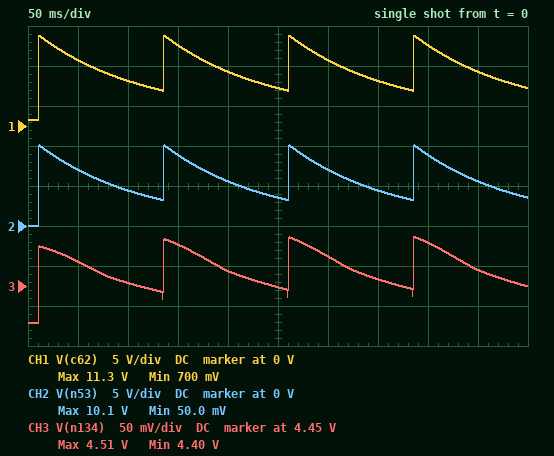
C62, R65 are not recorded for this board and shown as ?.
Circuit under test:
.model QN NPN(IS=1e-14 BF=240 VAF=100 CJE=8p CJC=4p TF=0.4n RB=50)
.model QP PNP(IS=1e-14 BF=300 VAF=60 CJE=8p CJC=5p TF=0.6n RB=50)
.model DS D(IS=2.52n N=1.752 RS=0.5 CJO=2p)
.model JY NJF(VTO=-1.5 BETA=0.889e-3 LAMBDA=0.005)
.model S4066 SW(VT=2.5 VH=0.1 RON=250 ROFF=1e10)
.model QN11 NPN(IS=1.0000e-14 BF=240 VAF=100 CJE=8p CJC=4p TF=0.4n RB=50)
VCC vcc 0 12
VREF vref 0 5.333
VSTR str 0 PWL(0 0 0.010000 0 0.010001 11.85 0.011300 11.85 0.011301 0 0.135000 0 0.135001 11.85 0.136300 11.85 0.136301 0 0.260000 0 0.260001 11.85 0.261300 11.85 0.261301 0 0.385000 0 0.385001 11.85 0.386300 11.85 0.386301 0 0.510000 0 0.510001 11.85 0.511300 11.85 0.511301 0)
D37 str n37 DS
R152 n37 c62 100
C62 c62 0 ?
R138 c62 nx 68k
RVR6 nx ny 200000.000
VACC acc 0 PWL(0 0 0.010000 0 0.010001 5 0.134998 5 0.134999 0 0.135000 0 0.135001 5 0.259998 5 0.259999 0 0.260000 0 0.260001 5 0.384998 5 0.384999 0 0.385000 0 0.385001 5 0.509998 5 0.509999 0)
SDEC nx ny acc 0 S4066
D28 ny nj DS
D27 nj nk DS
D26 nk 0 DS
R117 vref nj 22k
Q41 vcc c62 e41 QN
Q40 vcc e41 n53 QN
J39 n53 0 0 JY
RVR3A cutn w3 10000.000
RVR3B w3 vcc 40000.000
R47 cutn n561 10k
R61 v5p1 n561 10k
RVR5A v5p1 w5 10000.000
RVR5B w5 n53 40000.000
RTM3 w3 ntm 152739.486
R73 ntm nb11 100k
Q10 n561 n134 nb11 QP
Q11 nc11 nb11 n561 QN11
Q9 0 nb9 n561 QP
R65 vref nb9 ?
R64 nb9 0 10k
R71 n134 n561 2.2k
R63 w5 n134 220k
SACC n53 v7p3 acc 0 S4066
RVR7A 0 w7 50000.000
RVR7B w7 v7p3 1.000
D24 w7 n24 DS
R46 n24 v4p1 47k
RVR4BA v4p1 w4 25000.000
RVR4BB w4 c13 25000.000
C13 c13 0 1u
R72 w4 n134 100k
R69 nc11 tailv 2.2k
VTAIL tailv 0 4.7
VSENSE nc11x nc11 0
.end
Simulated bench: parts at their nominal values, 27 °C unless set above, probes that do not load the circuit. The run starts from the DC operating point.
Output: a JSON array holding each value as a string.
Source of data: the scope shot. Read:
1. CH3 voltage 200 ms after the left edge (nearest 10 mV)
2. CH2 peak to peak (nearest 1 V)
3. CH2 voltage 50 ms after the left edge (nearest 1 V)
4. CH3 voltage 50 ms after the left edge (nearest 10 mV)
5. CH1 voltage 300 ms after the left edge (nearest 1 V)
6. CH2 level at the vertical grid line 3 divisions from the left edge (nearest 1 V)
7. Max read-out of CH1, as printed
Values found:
["4.47 V", "10 V", "7 V", "4.48 V", "8 V", "9 V", "11.3 V"]
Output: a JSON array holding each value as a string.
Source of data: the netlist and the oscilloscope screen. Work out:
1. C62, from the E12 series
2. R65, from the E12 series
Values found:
["1.5 µF", "3.9 kΩ"]
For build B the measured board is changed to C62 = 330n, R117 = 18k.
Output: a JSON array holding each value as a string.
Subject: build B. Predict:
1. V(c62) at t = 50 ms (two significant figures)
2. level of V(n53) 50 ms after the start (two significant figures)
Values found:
["3.3 V", "2.1 V"]
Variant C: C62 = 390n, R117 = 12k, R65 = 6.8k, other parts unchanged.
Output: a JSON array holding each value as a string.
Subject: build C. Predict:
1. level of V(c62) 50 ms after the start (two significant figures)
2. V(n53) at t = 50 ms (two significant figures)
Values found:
["3.8 V", "2.6 V"]
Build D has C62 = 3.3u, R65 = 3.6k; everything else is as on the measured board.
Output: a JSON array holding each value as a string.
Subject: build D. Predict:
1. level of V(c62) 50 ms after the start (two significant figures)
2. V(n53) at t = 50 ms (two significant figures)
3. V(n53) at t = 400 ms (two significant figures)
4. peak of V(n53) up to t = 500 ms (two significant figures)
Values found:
["9.5 V", "8.3 V", "9.4 V", "9.9 V"]
